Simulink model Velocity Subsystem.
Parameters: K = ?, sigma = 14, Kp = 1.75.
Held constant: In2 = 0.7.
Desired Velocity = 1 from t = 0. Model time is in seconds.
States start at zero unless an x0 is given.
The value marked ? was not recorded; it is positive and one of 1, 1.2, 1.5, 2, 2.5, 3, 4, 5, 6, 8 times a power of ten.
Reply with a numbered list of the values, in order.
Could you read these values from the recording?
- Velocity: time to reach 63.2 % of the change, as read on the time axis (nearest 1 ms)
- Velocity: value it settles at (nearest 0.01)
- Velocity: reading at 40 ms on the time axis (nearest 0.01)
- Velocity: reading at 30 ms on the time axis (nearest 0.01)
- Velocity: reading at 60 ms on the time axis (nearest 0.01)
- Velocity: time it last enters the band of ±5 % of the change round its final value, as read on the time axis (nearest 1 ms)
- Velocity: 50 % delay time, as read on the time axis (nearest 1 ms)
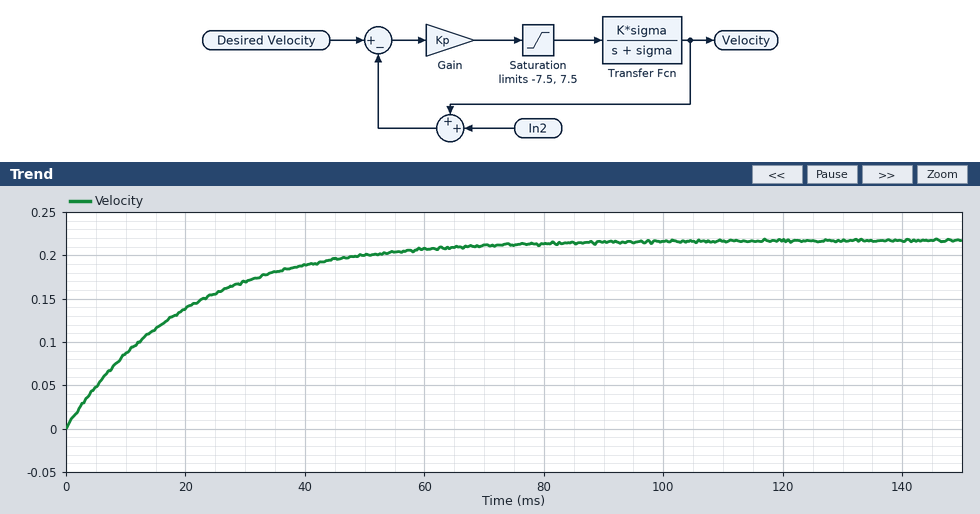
1. 20 ms
2. 0.22
3. 0.19
4. 0.17
5. 0.21
6. 59 ms
7. 14 ms
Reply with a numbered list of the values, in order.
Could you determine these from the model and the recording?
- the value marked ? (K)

1. 1.5
